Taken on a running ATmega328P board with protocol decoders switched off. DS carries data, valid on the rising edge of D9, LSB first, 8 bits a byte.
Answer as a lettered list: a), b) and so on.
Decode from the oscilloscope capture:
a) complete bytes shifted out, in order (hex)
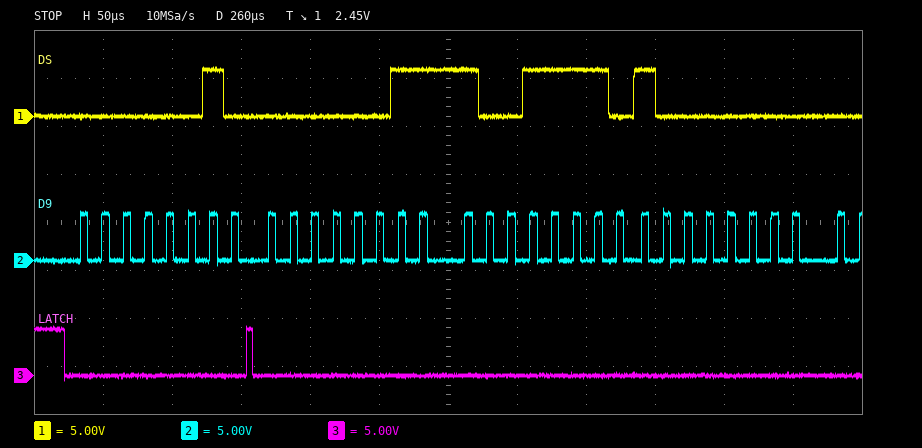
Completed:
a) 0x40 0xC0 0x79 0x01
